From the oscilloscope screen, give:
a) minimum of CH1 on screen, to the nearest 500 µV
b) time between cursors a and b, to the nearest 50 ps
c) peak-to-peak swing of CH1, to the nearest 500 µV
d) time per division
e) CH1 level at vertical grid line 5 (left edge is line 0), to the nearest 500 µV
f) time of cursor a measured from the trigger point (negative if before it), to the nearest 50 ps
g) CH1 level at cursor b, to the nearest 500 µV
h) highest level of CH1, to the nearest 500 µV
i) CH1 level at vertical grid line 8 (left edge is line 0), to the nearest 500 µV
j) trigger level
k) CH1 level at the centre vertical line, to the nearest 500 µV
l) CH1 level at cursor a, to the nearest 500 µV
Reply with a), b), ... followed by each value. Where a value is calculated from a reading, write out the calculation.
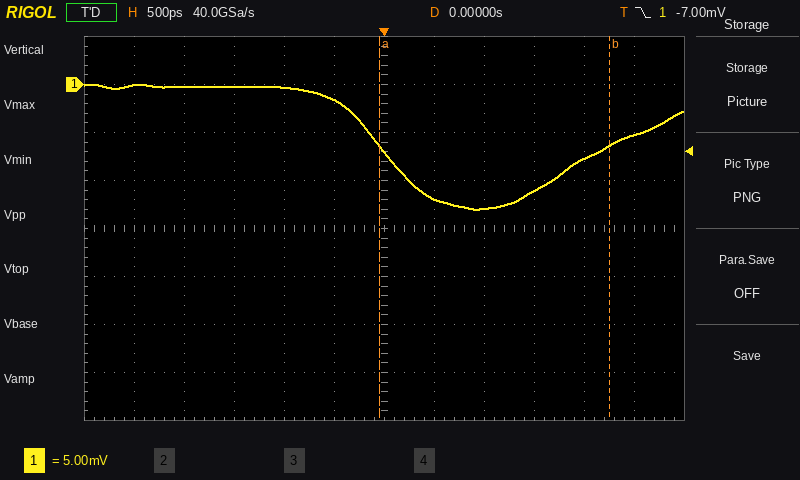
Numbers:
a) -13.0 mV
b) 2.30 ns
c) 0.0 mV − (-13.0 mV) = 13.0 mV
d) 500 ps
e) -1.5 mV
f) -50 ps
g) -6.5 mV
h) 0.0 mV
i) -13.0 mV
j) -7.00 mV
k) -7.0 mV
l) -6.5 mV
